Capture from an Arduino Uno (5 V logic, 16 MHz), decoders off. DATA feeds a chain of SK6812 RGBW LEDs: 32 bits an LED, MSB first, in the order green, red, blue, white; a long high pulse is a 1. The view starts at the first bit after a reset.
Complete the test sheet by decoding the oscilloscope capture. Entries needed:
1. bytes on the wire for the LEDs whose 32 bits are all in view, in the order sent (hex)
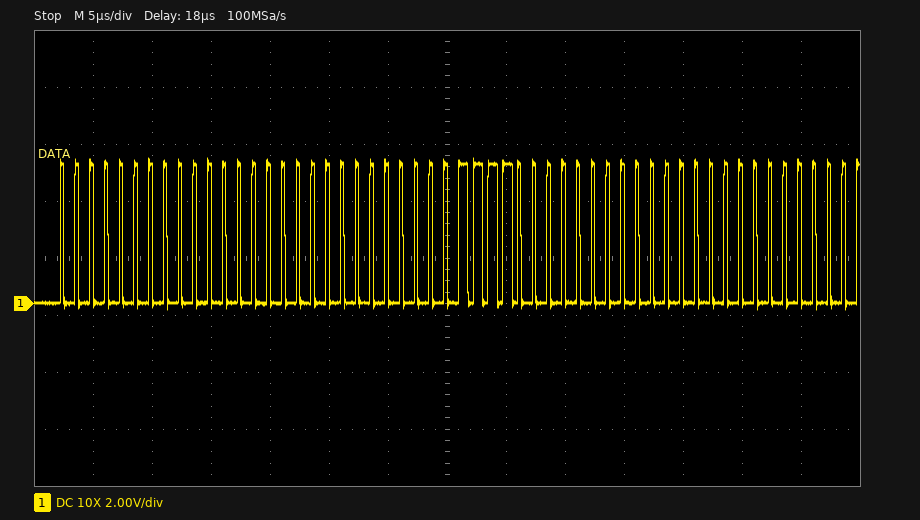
00 00 00 1E
